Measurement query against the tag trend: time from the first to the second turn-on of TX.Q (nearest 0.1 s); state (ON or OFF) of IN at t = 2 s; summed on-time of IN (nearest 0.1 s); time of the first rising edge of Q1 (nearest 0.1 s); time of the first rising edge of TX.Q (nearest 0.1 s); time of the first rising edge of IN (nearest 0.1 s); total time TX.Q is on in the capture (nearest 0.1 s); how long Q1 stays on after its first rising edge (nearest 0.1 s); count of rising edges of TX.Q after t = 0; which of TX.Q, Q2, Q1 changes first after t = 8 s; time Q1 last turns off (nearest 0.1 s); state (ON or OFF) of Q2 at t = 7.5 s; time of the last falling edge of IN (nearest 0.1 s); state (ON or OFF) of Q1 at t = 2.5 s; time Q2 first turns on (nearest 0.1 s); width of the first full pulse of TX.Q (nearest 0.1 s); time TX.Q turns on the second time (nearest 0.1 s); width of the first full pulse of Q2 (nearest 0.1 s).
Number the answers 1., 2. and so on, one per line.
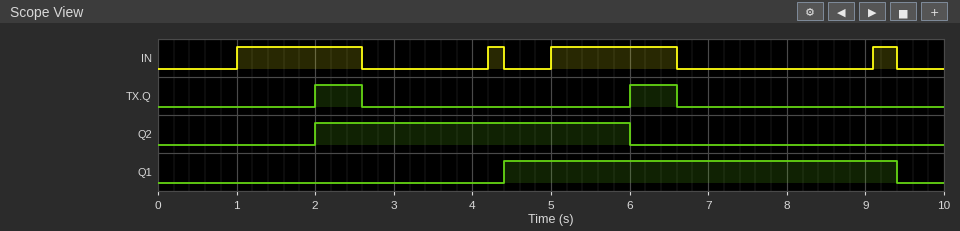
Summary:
1. 4.0 s
2. ON
3. 3.7 s
4. 4.4 s
5. 2.0 s
6. 1.0 s
7. 1.2 s
8. 5.0 s
9. 2
10. Q1
11. 9.4 s
12. OFF
13. 9.4 s
14. OFF
15. 2.0 s
16. 0.6 s
17. 6.0 s
18. 4.0 s
